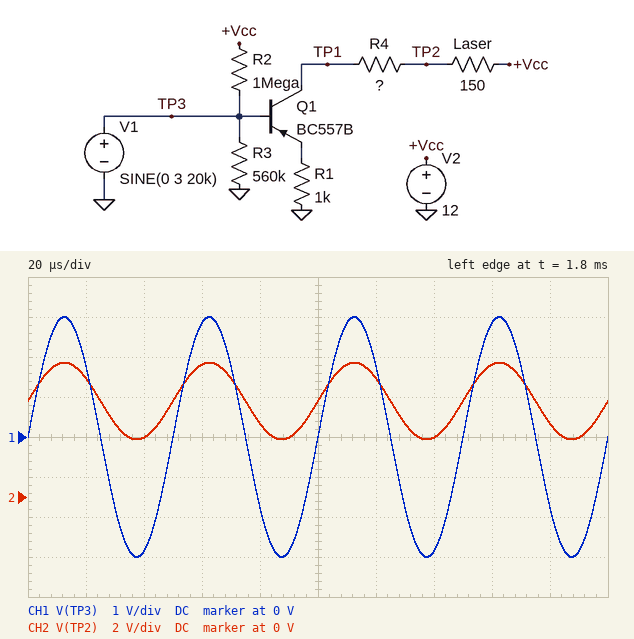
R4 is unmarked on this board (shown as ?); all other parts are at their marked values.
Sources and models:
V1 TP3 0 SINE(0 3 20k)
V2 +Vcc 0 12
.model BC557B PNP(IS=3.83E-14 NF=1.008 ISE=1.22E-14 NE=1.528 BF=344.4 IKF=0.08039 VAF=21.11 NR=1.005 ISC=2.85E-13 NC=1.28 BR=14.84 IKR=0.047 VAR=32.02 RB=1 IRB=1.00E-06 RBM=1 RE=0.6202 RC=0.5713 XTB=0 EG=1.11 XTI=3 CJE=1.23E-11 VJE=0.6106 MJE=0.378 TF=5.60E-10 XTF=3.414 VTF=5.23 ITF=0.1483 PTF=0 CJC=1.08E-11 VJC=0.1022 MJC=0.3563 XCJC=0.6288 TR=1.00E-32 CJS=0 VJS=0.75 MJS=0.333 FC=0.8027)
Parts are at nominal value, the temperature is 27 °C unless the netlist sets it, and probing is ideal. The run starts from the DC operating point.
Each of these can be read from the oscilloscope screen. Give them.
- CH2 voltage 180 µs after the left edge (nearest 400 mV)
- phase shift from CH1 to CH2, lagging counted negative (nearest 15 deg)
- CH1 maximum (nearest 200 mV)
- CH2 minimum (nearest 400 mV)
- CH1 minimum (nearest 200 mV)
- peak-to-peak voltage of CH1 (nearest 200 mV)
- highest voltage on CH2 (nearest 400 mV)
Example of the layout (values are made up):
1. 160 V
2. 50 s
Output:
1. 3.6 V
2. 0 deg
3. 3.0 V
4. 2.8 V
5. -3.0 V
6. 6.0 V
7. 6.8 V
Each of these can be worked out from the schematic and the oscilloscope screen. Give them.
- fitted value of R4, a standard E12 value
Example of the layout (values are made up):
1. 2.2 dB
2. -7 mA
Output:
1. 82 Ω
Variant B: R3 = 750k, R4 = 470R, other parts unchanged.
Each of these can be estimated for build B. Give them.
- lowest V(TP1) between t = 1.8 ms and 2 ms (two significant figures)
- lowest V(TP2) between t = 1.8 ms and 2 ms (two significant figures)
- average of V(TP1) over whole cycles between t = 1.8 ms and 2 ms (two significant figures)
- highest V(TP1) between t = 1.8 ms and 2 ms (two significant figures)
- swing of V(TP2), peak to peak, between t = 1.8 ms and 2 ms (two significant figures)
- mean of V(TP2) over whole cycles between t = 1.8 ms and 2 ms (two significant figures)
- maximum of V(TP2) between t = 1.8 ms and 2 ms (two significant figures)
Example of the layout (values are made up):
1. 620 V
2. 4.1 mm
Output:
1. -2.2 V
2. 8.6 V
3. 790 mV
4. 3.8 V
5. 1.4 V
6. 9.3 V
7. 10 V
